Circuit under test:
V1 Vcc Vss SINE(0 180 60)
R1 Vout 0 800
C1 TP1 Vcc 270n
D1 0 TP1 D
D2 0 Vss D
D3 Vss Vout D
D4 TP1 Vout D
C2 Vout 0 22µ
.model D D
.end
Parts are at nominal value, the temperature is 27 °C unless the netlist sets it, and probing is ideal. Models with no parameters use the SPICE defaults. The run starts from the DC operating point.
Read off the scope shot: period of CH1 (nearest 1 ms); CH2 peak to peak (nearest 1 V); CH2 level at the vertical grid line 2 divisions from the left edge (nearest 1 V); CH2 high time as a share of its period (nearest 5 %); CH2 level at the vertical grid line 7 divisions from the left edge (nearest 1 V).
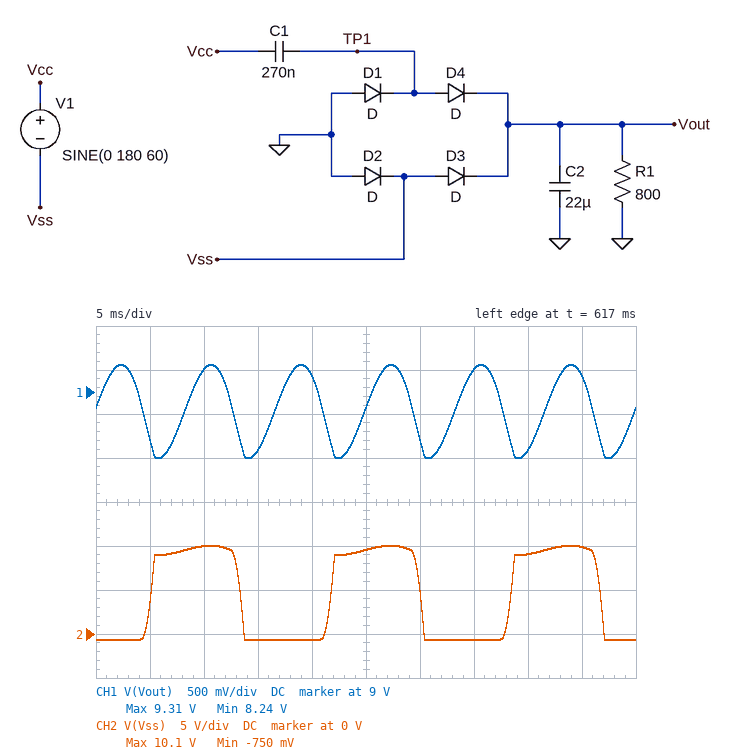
8 ms
11 V
10 V
50 %
-1 V
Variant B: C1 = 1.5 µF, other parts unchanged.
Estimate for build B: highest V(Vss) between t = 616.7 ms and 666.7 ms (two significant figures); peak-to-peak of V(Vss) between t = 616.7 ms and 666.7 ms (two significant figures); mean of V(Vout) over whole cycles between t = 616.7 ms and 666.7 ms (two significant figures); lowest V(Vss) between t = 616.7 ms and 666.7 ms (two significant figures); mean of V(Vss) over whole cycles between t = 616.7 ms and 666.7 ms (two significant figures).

43 V
44 V
40 V
-780 mV
20 V
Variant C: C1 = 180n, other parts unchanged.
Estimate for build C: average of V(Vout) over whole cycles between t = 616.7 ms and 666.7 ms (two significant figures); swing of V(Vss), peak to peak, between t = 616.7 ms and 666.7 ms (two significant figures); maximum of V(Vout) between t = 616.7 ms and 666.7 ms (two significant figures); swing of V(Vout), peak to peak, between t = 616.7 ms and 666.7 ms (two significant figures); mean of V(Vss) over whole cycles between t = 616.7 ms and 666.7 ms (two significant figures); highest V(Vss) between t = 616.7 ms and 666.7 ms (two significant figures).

6.0 V
7.7 V
6.3 V
680 mV
3.0 V
7.0 V
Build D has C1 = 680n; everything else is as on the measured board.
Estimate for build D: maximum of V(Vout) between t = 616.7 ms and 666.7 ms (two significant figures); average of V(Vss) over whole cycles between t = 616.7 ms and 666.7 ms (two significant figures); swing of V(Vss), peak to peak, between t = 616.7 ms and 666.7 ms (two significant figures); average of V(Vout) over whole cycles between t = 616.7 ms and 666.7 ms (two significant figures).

22 V
10 V
23 V
21 V
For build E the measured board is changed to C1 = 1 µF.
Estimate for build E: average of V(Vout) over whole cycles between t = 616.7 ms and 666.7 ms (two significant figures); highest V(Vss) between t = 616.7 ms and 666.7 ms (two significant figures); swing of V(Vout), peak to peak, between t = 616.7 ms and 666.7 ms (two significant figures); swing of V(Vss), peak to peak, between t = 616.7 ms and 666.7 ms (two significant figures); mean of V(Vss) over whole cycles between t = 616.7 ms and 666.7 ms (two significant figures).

29 V
31 V
4.7 V
32 V
14 V
